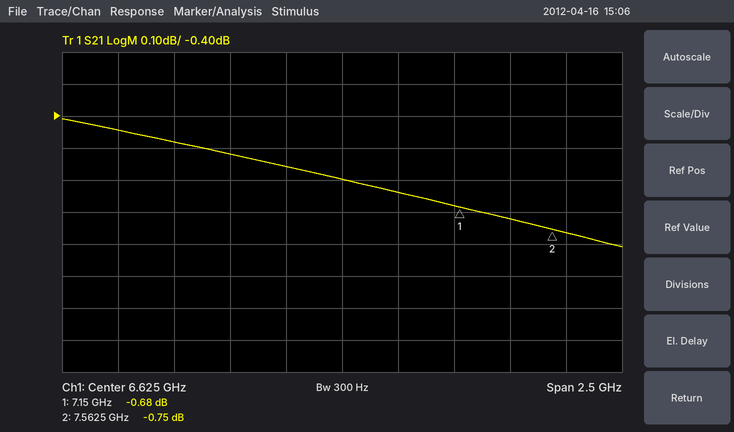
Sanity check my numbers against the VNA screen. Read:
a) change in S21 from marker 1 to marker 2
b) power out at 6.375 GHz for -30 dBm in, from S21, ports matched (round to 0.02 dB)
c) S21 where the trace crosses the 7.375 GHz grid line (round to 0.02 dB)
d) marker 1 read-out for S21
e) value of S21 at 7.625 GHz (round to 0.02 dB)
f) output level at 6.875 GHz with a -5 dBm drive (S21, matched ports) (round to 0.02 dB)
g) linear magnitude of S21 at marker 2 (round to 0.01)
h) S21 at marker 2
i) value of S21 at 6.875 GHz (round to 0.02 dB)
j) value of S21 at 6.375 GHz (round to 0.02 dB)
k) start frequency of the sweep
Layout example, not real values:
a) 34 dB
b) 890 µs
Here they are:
a) -0.07 dB
b) -30.56 dBm
c) -0.72 dB
d) -0.68 dB
e) -0.76 dB
f) -5.64 dBm
g) 0.92
h) -0.75 dB
i) -0.64 dB
j) -0.56 dB
k) 5.375 GHz
